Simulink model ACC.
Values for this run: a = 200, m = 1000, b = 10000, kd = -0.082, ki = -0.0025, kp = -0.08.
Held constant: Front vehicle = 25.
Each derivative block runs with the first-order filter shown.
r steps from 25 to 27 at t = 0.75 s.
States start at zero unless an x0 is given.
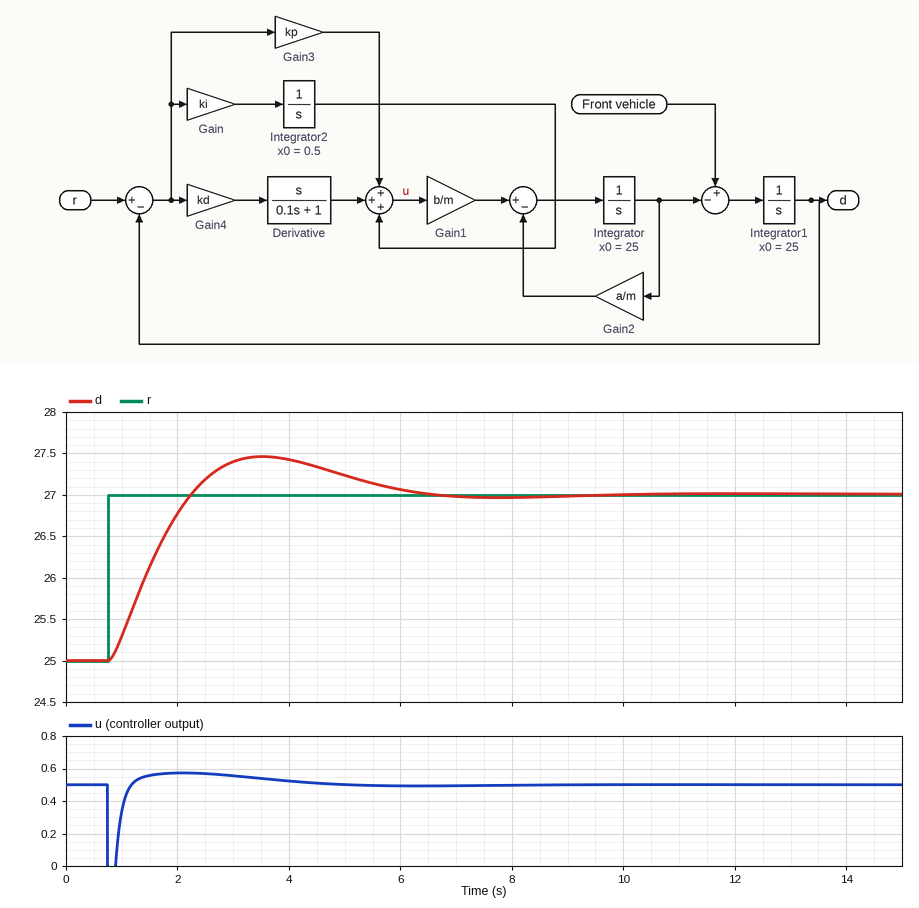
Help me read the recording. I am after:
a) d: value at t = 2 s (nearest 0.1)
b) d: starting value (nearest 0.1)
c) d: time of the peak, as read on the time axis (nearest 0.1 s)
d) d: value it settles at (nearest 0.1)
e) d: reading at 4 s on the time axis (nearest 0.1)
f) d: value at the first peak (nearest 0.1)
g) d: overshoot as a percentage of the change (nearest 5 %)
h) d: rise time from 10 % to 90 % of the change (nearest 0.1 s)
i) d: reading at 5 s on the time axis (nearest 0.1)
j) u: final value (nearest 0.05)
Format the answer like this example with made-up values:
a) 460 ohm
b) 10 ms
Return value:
a) 26.8
b) 25.0
c) 3.5 s
d) 27.0
e) 27.4
f) 27.5
g) 25 %
h) 1.1 s
i) 27.2
j) 0.50
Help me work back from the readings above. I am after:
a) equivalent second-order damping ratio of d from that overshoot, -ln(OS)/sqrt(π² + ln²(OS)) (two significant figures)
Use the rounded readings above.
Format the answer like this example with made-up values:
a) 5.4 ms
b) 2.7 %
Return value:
a) 0.40
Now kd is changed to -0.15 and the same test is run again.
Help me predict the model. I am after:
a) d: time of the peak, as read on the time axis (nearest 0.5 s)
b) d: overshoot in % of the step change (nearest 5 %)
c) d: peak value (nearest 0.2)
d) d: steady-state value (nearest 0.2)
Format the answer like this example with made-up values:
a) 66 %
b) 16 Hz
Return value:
a) 3.0 s
b) 10 %
c) 27.2
d) 27.0
